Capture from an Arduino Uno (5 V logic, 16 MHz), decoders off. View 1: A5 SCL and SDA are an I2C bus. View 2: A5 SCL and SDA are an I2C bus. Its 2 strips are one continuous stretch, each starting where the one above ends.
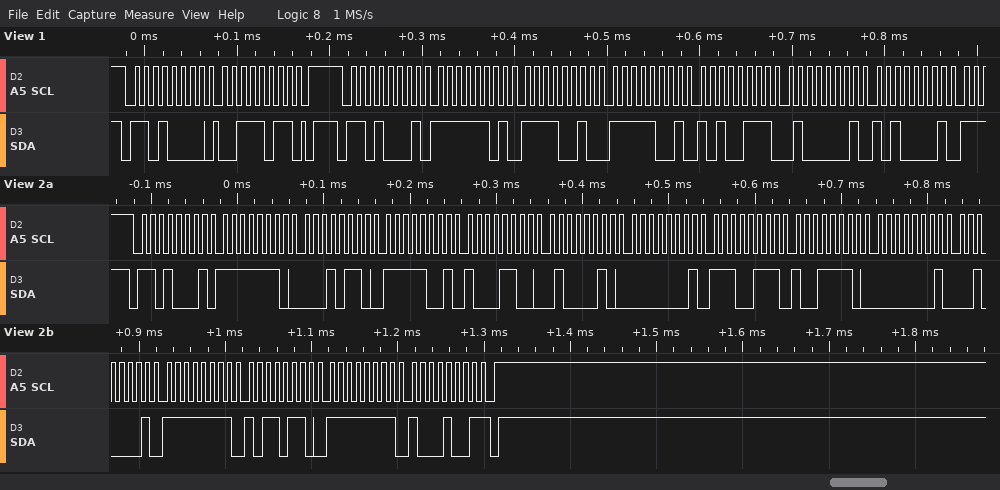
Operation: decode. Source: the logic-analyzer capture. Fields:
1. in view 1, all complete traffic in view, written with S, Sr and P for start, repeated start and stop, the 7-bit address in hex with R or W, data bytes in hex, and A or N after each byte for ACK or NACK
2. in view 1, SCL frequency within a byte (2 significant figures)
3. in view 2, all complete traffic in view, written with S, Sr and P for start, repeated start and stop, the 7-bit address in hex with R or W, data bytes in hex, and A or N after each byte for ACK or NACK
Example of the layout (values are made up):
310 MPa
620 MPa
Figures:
S 68W A 3B A P S 68R A FD A F2 A F9 A A7 A 41 A A1 A
100 kHz
S 68R A FE A 16 A F9 A 8C A 42 A 01 A E7 A 9E A 01 A 21 A FF A B6 A FF A 89 N P
